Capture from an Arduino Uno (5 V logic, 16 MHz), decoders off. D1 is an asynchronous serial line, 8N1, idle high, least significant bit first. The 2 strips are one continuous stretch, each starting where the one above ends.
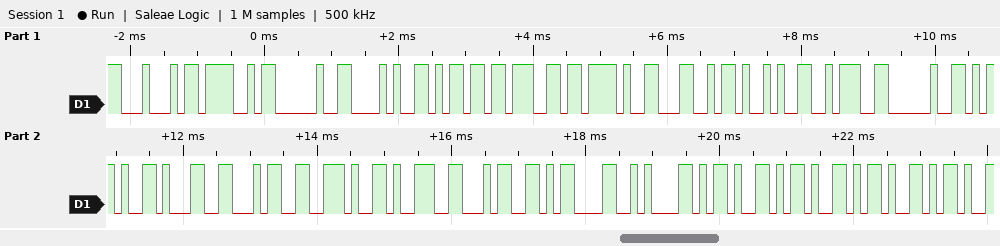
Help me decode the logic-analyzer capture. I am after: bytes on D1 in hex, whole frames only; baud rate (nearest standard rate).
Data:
44 4F 20 28 6D 67 2F 4C 29 3A 20 2D 31 34 2E 39 34 0D 0A 2D 2D 2D 2D
9600 baud
